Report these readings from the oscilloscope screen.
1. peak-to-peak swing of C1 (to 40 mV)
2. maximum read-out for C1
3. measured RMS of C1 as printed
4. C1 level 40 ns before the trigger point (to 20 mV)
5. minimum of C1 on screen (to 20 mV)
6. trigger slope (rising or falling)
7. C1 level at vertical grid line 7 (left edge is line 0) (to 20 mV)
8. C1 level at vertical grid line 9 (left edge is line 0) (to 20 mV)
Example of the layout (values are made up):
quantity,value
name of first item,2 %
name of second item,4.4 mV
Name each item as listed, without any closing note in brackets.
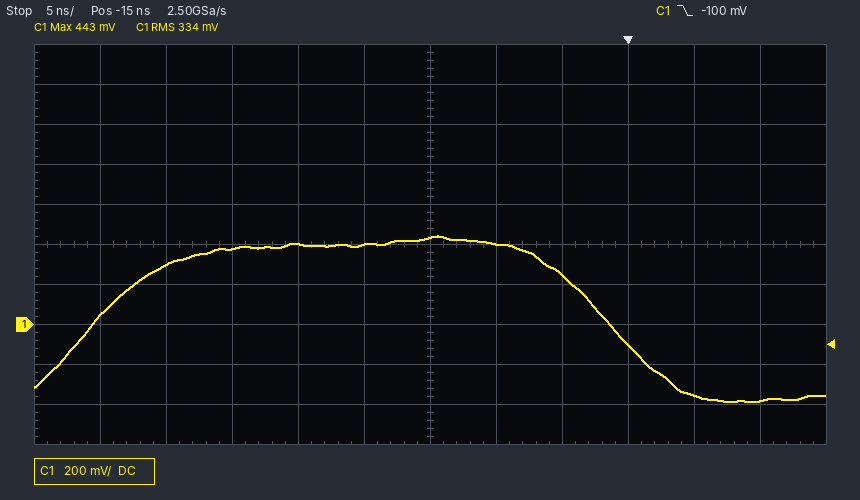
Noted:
quantity,value
peak-to-peak swing of C1,840 mV
maximum read-out for C1,443 mV
measured RMS of C1 as printed,334 mV
C1 level 40 ns before the trigger point,40 mV
minimum of C1 on screen,-380 mV
trigger slope,falling
C1 level at vertical grid line 7 (left edge is line 0),400 mV
C1 level at vertical grid line 9 (left edge is line 0),-100 mV
